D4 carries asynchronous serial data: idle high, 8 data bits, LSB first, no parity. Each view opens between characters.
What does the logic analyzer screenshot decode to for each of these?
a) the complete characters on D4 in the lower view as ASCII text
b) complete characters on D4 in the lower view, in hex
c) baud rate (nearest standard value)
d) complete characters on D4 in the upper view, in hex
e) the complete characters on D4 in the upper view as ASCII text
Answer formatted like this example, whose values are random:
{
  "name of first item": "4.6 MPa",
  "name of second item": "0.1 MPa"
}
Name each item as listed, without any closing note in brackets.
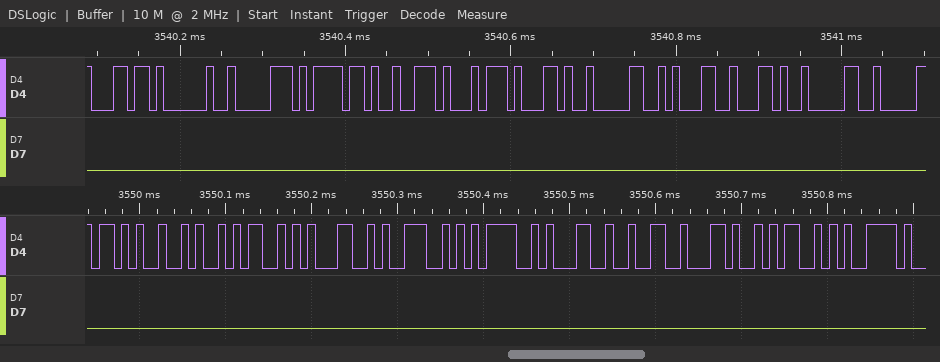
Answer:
{
  "the complete characters on D4 in the lower view as ASCII text": "\"+JSLN=12,My\"",
  "complete characters on D4 in the lower view, in hex": "2B, 4A, 53, 4C, 4E, 3D, 31, 32, 2C, 4D, 79",
  "baud rate": "115200 baud",
  "complete characters on D4 in the upper view, in hex": "6C, 20, 70, 6F, 72, 74, 2C, 30, 31, 2C, 30",
  "the complete characters on D4 in the upper view as ASCII text": "\"l port,01,0\""
}
